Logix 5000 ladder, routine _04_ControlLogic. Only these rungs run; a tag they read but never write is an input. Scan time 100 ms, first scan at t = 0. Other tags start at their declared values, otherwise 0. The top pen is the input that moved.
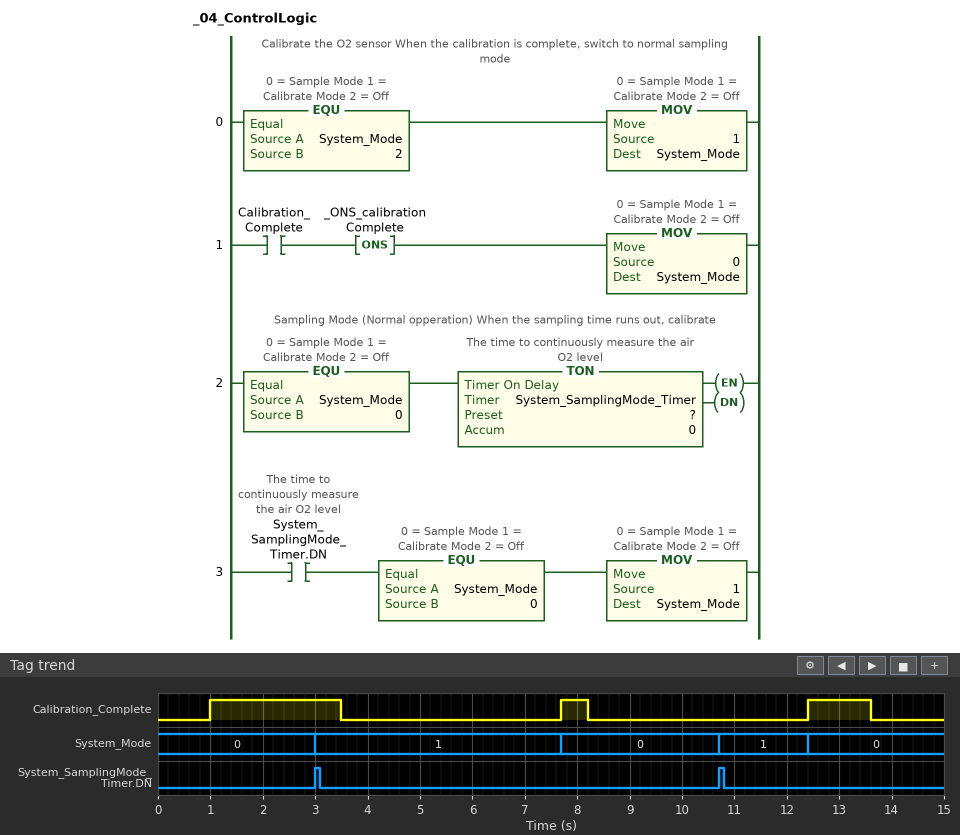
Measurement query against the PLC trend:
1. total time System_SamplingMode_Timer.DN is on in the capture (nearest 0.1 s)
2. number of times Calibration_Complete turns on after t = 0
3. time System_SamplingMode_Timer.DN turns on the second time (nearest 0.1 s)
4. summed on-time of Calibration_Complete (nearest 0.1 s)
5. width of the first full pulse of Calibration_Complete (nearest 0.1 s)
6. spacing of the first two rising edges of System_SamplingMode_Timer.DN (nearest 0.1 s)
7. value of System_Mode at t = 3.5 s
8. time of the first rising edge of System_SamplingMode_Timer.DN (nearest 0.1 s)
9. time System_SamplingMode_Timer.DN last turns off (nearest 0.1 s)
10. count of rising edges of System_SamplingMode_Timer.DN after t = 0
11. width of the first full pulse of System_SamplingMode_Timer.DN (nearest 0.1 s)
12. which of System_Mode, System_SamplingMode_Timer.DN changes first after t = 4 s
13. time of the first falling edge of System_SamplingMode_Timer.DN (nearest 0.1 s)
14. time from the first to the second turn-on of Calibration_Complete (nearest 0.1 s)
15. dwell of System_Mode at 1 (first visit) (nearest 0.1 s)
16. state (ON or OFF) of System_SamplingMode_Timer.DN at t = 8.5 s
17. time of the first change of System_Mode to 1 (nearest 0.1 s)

0.2 s
3
10.7 s
4.2 s
2.5 s
7.7 s
1
3.0 s
10.8 s
2
0.1 s
System_Mode
3.1 s
6.7 s
4.7 s
OFF
3.0 s
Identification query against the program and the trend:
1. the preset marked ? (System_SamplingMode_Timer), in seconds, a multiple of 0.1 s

3.0 s
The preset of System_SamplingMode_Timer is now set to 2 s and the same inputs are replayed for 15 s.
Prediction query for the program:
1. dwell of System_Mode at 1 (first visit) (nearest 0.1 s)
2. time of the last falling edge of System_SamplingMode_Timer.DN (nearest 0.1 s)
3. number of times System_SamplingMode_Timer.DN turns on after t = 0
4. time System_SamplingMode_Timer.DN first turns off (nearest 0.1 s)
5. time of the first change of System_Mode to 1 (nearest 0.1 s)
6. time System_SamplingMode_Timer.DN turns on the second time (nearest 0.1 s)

5.7 s
14.5 s
3
2.1 s
2.0 s
9.7 s
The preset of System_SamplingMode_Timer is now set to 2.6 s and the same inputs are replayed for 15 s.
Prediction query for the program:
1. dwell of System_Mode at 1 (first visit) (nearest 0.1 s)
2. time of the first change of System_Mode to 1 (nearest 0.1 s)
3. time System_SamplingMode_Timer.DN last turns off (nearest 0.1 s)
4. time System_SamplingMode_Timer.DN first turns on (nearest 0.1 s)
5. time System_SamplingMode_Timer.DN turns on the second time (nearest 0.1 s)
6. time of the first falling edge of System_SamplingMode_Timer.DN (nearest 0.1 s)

5.1 s
2.6 s
10.4 s
2.6 s
10.3 s
2.7 s
